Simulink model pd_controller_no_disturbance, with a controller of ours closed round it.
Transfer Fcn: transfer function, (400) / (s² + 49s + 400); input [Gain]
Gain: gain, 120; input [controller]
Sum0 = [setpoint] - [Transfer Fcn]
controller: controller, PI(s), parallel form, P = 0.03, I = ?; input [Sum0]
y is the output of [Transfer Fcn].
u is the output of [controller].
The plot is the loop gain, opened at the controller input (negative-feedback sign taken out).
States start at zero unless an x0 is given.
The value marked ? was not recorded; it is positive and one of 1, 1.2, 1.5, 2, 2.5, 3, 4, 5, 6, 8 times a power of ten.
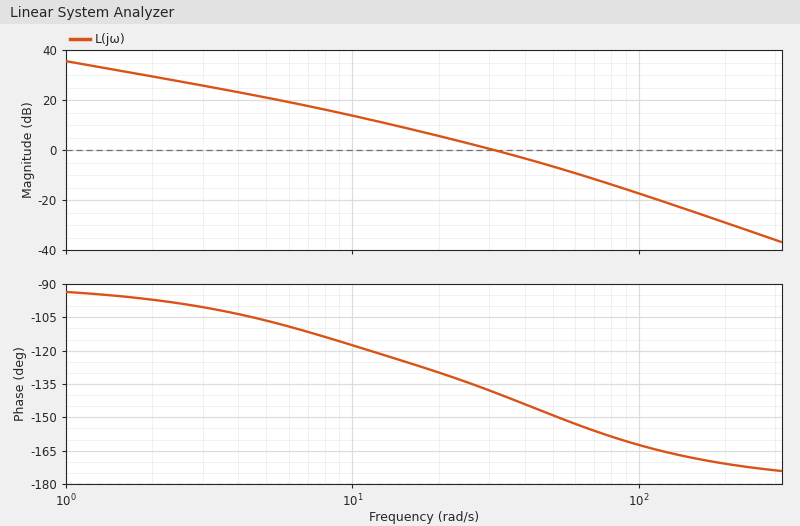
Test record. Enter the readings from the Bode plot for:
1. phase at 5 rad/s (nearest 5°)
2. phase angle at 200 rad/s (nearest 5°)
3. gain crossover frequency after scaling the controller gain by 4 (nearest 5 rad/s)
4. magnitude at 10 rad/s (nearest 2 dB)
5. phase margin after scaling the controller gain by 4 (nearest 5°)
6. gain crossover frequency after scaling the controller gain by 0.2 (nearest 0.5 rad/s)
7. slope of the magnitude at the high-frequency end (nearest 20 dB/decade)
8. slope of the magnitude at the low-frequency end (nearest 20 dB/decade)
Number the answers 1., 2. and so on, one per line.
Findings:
1. -105°
2. -170°
3. 70 rad/s
4. 14 dB
5. 25°
6. 10.0 rad/s
7. -40 dB/decade
8. -20 dB/decade
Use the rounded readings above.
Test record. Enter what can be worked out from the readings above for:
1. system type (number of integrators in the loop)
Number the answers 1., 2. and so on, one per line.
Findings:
1. 1
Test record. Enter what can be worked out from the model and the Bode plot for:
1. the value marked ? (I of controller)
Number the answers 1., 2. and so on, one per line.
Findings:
1. 0.5
